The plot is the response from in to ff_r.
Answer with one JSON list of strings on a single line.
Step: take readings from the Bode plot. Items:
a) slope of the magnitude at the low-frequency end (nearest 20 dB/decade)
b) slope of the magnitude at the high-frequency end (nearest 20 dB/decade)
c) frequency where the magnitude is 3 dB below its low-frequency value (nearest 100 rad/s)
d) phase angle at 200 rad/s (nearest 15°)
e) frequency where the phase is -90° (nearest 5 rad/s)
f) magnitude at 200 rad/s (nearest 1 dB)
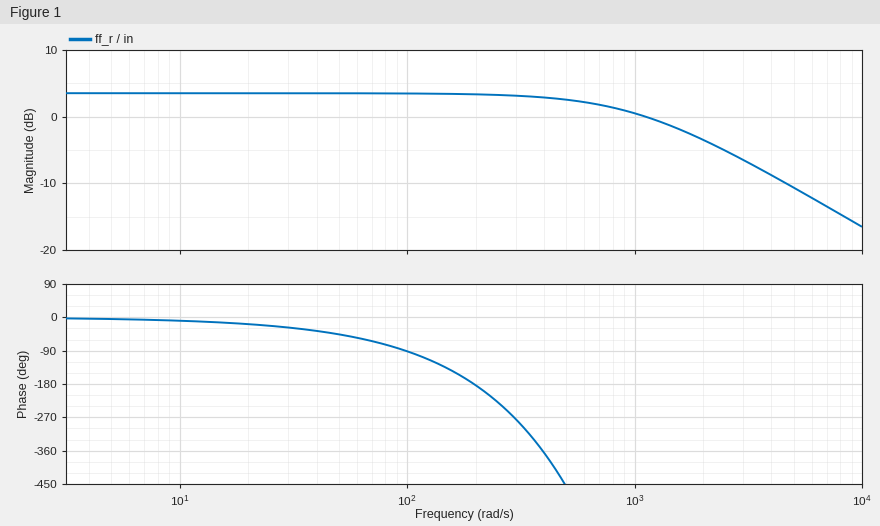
["0 dB/decade", "-20 dB/decade", "1000 rad/s", "-180°", "100 rad/s", "3 dB"]
